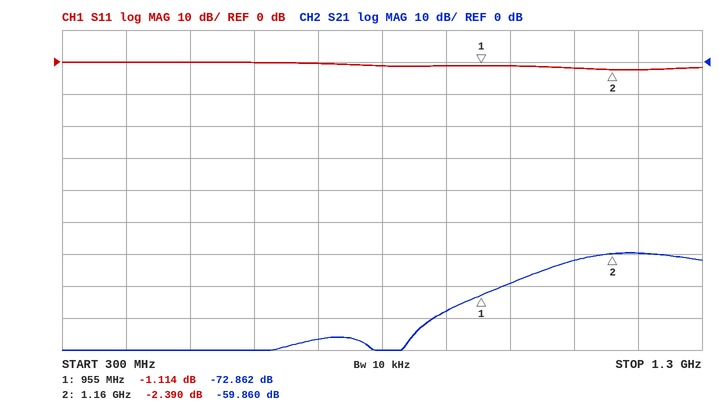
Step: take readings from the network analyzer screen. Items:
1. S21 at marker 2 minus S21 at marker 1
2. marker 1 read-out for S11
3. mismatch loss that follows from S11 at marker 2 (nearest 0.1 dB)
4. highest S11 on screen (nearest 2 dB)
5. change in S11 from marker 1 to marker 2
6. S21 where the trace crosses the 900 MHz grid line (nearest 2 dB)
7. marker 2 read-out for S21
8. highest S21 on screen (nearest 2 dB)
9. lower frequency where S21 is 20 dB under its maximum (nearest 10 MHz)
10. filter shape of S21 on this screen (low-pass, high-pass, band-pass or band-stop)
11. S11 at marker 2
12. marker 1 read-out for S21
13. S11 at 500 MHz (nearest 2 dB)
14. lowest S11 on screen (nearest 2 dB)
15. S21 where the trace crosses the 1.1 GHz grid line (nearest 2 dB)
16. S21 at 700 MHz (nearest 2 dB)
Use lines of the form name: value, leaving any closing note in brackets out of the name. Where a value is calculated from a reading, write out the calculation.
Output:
S21 at marker 2 minus S21 at marker 1: -59.86 − (-72.862) = 13.002 dB
marker 1 read-out for S11: -1.114 dB
mismatch loss that follows from S11 at marker 2: −10 log10(1 − 10^(-2.39/10)) ≈ 3.7 dB
highest S11 on screen: 0 dB
change in S11 from marker 1 to marker 2: -2.39 − (-1.114) = -1.276 dB
S21 where the trace crosses the 900 MHz grid line: -78 dB
marker 2 read-out for S21: -59.860 dB
highest S21 on screen: -60 dB
lower frequency where S21 is 20 dB under its maximum: 880 MHz
filter shape of S21 on this screen: high-pass
S11 at marker 2: -2.390 dB
marker 1 read-out for S21: -72.862 dB
S11 at 500 MHz: 0 dB
lowest S11 on screen: -2 dB
S21 where the trace crosses the 1.1 GHz grid line: -62 dB
S21 at 700 MHz: -86 dB
